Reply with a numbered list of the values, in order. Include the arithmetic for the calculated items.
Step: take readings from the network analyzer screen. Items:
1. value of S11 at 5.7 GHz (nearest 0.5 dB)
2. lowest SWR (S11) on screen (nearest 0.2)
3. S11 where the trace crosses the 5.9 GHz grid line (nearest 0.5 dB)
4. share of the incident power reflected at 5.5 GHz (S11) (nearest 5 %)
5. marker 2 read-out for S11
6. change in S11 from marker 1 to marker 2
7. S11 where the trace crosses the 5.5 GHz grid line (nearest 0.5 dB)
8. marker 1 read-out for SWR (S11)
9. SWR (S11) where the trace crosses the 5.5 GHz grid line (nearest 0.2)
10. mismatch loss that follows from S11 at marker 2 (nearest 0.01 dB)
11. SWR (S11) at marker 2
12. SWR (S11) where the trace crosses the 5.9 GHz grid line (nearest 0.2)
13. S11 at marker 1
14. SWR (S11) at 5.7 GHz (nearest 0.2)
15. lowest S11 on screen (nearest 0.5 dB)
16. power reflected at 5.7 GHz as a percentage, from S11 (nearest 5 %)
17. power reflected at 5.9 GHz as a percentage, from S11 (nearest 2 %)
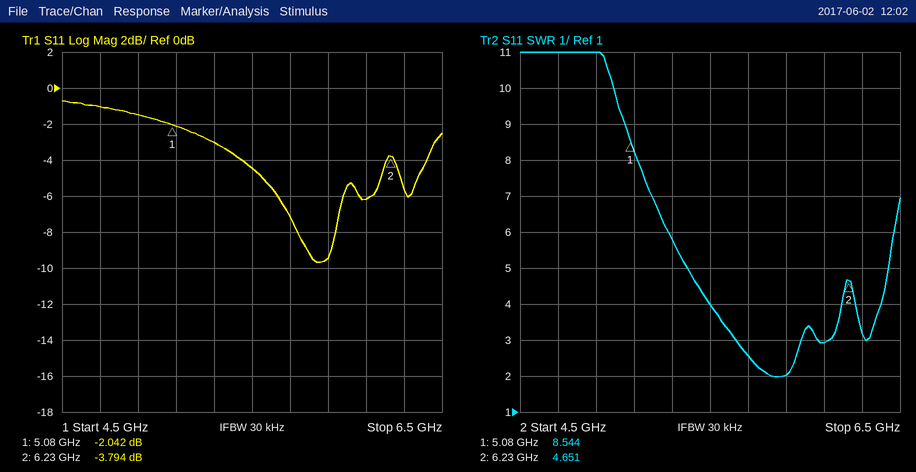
1. -7.0 dB
2. 2.0
3. -9.5 dB
4. 10^(-4.5/10) ≈ 35 %
5. -3.794 dB
6. -3.794 − (-2.042) = -1.752 dB
7. -4.5 dB
8. 8.544
9. 4.0
10. −10 log10(1 − 10^(-3.794/10)) ≈ 2.35 dB
11. 4.651
12. 2.0
13. -2.042 dB
14. 2.6
15. -9.5 dB
16. 10^(-7/10) ≈ 20 %
17. 10^(-9.5/10) ≈ 11.2 %, so 12 % to the nearest 2 %
